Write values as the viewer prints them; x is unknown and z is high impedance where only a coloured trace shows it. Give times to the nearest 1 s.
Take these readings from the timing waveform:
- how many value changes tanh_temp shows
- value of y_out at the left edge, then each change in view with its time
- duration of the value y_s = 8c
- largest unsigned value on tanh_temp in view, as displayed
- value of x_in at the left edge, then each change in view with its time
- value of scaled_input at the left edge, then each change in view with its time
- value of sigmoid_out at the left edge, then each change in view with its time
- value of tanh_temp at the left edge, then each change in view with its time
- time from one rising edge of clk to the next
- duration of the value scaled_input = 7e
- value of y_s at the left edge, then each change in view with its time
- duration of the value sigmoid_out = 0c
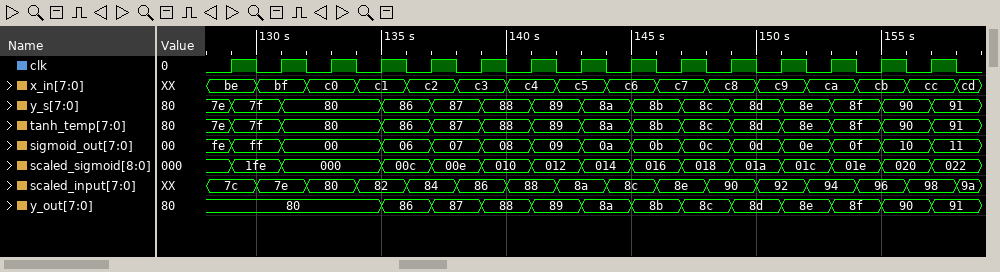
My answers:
14
80, 86 at 135 s, 87 at 137 s, 88 at 139 s, 89 at 141 s, 8a at 143 s, 8b at 145 s, 8c at 147 s, 8d at 149 s, 8e at 151 s, 8f at 153 s, 90 at 155 s, 91 at 157 s
2 s
91
be, bf at 130 s, c0 at 132 s, c1 at 134 s, c2 at 136 s, c3 at 138 s, c4 at 140 s, c5 at 142 s, c6 at 144 s, c7 at 146 s, c8 at 148 s, c9 at 150 s, ca at 152 s, cb at 154 s, cc at 156 s, cd at 158 s
7c, 7e at 130 s, 80 at 132 s, 82 at 134 s, 84 at 136 s, 86 at 138 s, 88 at 140 s, 8a at 142 s, 8c at 144 s, 8e at 146 s, 90 at 148 s, 92 at 150 s, 94 at 152 s, 96 at 154 s, 98 at 156 s, 9a at 158 s
fe, ff at 129 s, 00 at 131 s, 06 at 135 s, 07 at 137 s, 08 at 139 s, 09 at 141 s, 0a at 143 s, 0b at 145 s, 0c at 147 s, 0d at 149 s, 0e at 151 s, 0f at 153 s, 10 at 155 s, 11 at 157 s
7e, 7f at 129 s, 80 at 131 s, 86 at 135 s, 87 at 137 s, 88 at 139 s, 89 at 141 s, 8a at 143 s, 8b at 145 s, 8c at 147 s, 8d at 149 s, 8e at 151 s, 8f at 153 s, 90 at 155 s, 91 at 157 s
2 s
2 s
7e, 7f at 129 s, 80 at 131 s, 86 at 135 s, 87 at 137 s, 88 at 139 s, 89 at 141 s, 8a at 143 s, 8b at 145 s, 8c at 147 s, 8d at 149 s, 8e at 151 s, 8f at 153 s, 90 at 155 s, 91 at 157 s
2 s
